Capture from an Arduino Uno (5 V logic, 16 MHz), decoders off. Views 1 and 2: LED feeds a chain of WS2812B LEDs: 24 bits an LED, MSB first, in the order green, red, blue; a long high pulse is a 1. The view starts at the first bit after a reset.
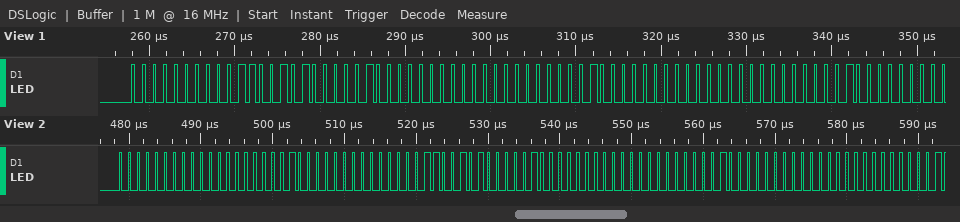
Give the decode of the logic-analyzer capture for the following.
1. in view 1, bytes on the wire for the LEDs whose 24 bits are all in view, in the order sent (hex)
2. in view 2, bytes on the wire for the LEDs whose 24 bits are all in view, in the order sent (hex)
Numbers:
00 32 82 00 00 10 00 00 10
00 00 10 00 32 82 00 00 10
